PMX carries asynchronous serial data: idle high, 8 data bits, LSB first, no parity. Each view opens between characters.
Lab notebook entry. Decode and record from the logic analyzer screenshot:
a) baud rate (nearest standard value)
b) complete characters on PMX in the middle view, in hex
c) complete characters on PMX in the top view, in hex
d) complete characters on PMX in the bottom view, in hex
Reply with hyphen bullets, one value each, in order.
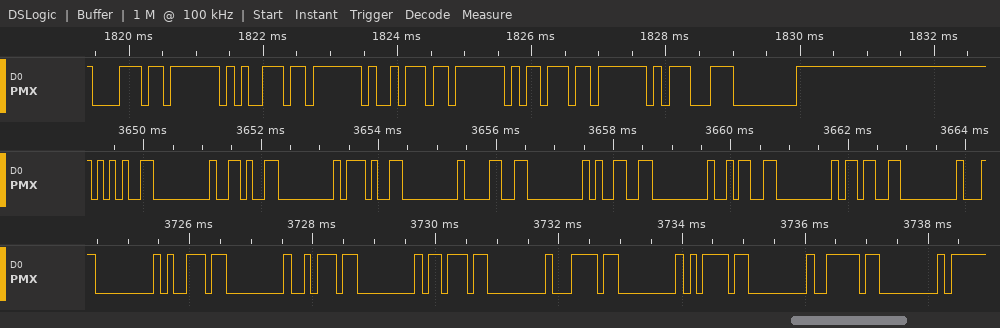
- 9600 baud
- 95, 00, 96, 00, 97, 00, 98, 00, 99, 00, 9A, 00, 9B, 00
- B8, 7F, B9, 7F, BA, 7F, BB, 7F, C7, 00
- 00, B9, 00, BA, 00, BB, 00, BC, 00, BD, 00, BE, 00
